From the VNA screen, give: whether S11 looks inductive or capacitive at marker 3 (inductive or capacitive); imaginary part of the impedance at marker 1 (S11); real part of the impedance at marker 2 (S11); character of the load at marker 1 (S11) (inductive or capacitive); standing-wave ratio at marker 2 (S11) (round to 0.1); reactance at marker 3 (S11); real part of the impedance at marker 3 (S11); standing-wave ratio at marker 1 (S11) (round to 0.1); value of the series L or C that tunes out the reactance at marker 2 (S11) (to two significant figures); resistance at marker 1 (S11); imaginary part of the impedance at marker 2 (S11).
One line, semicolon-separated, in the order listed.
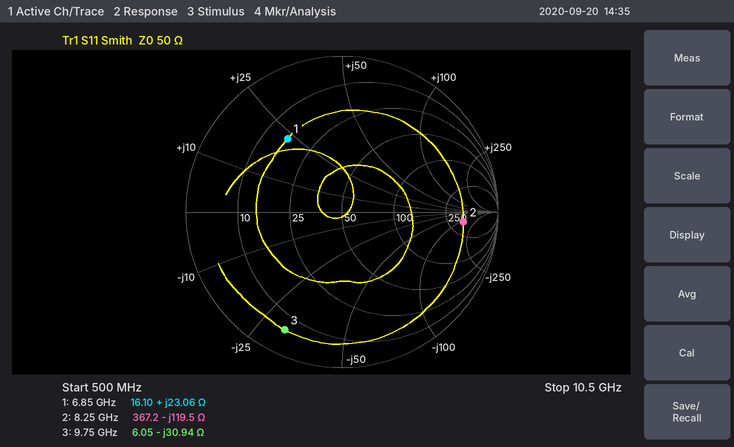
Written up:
capacitive; +23.06 Ω; 367.2 Ω; inductive; 8.1; -30.94 Ω; 6.05 Ω; 3.8; 2.3 nH; 16.10 Ω; -119.5 Ω
